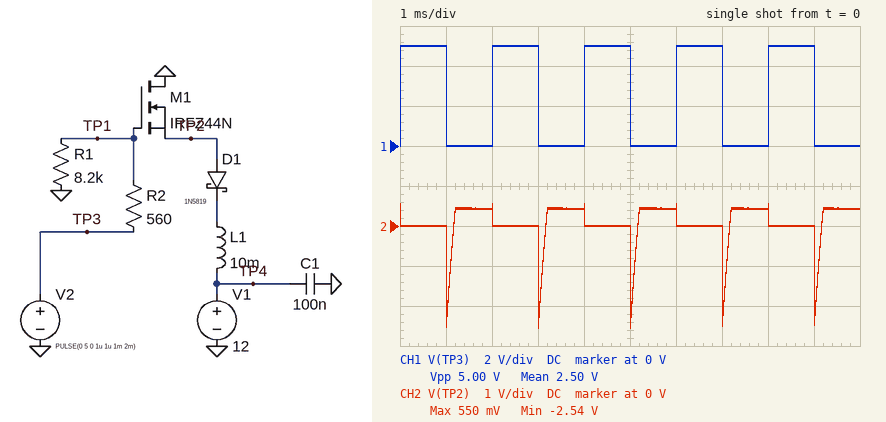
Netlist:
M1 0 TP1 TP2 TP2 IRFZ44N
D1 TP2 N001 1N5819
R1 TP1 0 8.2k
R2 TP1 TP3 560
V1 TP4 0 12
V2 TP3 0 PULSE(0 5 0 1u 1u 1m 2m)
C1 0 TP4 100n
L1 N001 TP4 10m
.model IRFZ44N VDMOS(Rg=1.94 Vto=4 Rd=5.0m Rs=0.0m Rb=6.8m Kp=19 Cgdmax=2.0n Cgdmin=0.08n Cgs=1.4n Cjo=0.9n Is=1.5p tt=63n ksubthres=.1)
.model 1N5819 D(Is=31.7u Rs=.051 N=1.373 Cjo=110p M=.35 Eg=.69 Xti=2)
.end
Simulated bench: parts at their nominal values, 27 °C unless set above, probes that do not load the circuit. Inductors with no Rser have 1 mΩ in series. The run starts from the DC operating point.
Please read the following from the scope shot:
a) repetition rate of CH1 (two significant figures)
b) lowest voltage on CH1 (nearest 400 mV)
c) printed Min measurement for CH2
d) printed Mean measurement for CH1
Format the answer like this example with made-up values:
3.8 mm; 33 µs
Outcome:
500 Hz; 0 V; -2.54 V; 2.50 V
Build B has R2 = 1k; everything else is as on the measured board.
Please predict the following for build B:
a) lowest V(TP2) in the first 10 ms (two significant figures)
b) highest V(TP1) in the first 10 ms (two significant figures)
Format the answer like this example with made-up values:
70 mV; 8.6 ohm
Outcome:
-2.4 V; 4.5 V
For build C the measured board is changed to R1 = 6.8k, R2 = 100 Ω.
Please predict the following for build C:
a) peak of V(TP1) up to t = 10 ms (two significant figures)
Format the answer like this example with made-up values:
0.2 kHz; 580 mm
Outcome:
4.9 V
